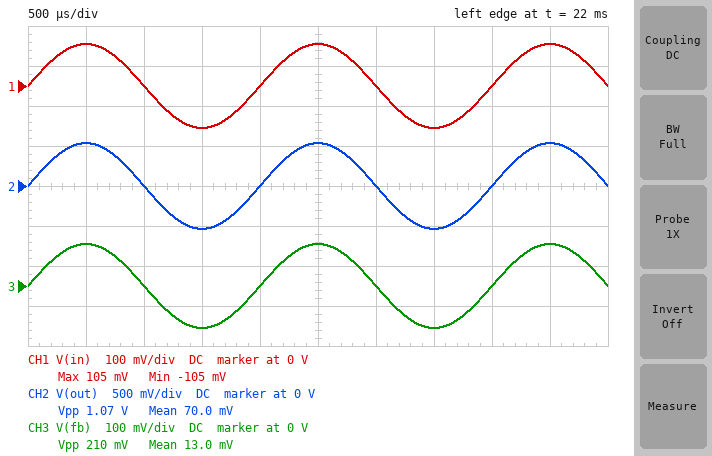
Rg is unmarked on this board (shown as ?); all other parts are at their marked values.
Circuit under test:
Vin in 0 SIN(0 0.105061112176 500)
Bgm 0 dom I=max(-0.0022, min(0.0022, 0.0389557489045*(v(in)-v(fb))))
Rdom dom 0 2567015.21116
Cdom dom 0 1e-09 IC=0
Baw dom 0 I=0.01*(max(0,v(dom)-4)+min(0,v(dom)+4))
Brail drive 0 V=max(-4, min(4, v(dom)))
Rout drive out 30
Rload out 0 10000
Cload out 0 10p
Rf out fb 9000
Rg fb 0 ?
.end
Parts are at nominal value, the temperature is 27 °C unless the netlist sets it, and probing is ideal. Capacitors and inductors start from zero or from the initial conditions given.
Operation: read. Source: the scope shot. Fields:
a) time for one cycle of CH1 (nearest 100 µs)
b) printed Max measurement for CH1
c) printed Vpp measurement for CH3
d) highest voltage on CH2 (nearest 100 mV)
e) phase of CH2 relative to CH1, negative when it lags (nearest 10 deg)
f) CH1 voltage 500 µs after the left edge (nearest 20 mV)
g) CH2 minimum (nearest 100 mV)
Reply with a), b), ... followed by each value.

a) 2.0 ms
b) 105 mV
c) 210 mV
d) 500 mV
e) 0 deg
f) 100 mV
g) -500 mV
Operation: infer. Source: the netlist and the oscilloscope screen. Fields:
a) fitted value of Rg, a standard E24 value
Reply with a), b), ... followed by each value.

a) 2.2 kΩ
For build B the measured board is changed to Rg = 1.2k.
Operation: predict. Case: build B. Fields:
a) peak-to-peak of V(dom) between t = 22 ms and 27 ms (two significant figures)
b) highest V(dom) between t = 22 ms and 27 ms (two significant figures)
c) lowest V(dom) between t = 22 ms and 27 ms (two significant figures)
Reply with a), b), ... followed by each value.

a) 1.8 V
b) 900 mV
c) -900 mV
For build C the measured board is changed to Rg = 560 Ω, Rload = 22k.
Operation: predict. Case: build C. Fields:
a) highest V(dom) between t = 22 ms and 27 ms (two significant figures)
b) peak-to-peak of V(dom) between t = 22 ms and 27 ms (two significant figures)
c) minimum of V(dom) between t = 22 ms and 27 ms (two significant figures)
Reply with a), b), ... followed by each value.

a) 1.8 V
b) 3.6 V
c) -1.8 V
